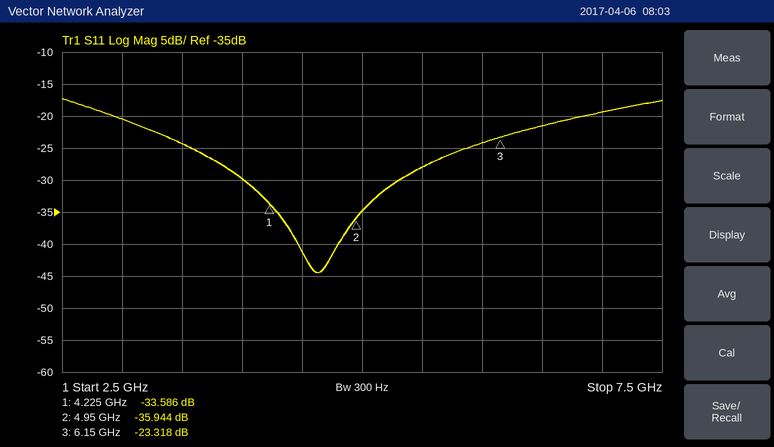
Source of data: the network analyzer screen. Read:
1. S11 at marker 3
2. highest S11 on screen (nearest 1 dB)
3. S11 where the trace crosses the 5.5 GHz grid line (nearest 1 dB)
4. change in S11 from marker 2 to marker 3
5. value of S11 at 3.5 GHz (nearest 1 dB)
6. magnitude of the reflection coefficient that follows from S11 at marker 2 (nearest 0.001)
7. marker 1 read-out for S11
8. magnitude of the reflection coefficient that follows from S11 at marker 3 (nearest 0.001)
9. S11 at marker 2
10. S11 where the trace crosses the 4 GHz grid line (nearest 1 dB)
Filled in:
-23.318 dB
-17 dB
-28 dB
12.626 dB
-24 dB
0.016
-33.586 dB
0.068
-35.944 dB
-30 dB
